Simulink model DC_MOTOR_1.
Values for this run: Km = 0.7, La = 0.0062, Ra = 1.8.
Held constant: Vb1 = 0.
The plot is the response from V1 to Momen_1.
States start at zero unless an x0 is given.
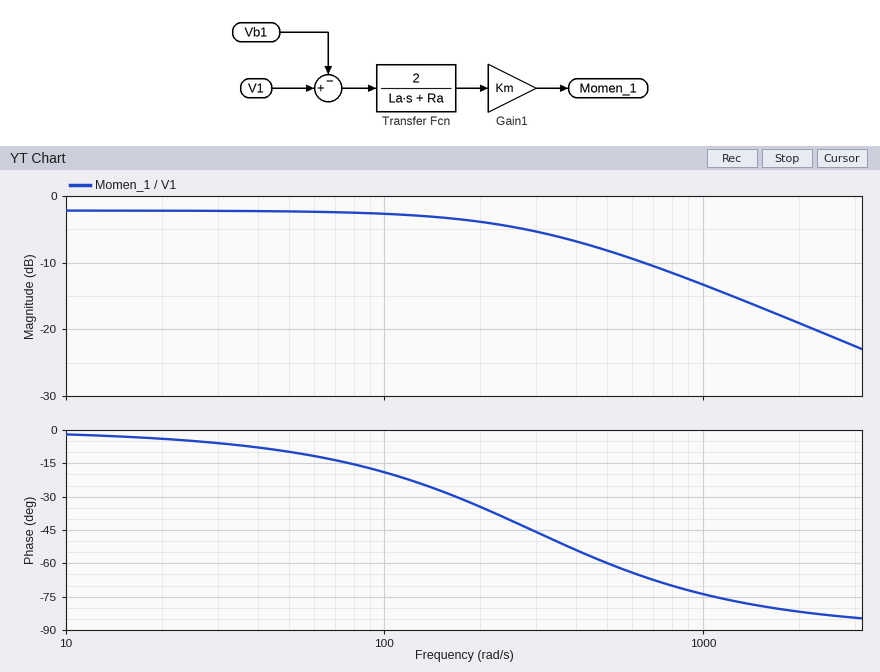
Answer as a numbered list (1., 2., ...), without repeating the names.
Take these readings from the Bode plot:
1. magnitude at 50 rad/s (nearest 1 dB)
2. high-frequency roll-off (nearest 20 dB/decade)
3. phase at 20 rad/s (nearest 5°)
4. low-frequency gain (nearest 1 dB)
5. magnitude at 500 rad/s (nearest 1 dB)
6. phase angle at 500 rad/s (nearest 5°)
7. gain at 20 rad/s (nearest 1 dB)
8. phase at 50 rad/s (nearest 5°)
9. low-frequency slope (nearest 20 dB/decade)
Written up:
1. -2 dB
2. -20 dB/decade
3. -5°
4. -2 dB
5. -8 dB
6. -60°
7. -2 dB
8. -10°
9. 0 dB/decade
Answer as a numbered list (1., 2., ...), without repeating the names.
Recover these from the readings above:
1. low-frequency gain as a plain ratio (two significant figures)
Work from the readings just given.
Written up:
1. 0.79
